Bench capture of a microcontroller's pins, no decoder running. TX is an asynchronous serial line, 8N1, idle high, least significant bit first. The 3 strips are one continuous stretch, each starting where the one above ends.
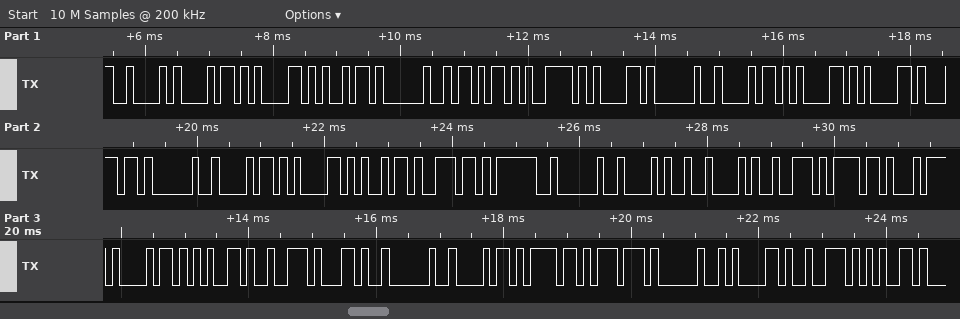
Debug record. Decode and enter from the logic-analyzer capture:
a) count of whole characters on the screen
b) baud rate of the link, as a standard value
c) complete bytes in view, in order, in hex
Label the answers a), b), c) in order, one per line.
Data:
a) 37
b) 9600 baud
c) 42 68 61 69 20 6B 79 61 20 68 61 61 6C 20 68 61 69 6E 3F 20 28 42 72 6F 74 68 65 72 2C 20 68 6F 77 20 61 72 65
